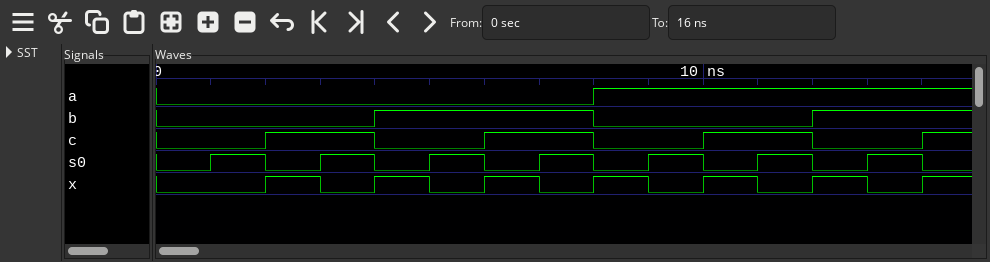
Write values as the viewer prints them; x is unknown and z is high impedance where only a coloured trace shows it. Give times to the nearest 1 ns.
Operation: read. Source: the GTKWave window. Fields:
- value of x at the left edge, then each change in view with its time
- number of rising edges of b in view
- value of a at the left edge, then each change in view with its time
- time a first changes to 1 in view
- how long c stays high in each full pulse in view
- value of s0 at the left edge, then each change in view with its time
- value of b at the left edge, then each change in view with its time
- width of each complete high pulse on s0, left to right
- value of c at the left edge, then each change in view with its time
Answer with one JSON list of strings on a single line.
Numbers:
["0, 1 at 2 ns, 0 at 3 ns, 1 at 4 ns, 0 at 5 ns, 1 at 6 ns, 0 at 7 ns, 1 at 8 ns, 0 at 9 ns, 1 at 10 ns, 0 at 11 ns, 1 at 12 ns, 0 at 13 ns, 1 at 14 ns", "2", "0, 1 at 8 ns", "8 ns", "2 ns, 2 ns, 2 ns", "0, 1 at 1 ns, 0 at 2 ns, 1 at 3 ns, 0 at 4 ns, 1 at 5 ns, 0 at 6 ns, 1 at 7 ns, 0 at 8 ns, 1 at 9 ns, 0 at 10 ns, 1 at 11 ns, 0 at 12 ns, 1 at 13 ns, 0 at 14 ns", "0, 1 at 4 ns, 0 at 8 ns, 1 at 12 ns", "1 ns, 1 ns, 1 ns, 1 ns, 1 ns, 1 ns, 1 ns", "0, 1 at 2 ns, 0 at 4 ns, 1 at 6 ns, 0 at 8 ns, 1 at 10 ns, 0 at 12 ns, 1 at 14 ns"]
